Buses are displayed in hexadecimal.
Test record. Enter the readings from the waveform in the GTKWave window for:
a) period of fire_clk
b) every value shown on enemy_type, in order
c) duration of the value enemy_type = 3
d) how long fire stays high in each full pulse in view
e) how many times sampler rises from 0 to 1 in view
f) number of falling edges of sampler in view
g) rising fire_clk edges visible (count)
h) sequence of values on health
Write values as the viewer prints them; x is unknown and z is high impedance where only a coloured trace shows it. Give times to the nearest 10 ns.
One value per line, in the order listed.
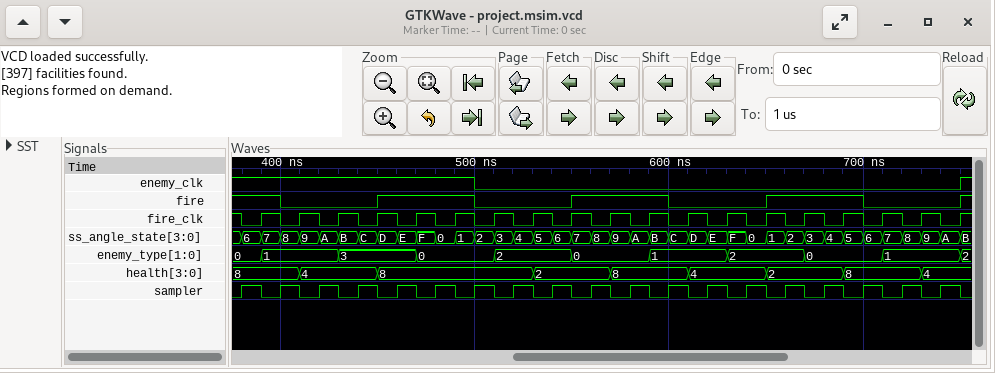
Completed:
20 ns
0, 1, 3, 0, 2, 0, 1, 2, 0, 1, 2
40 ns
50 ns, 50 ns, 50 ns
19
19
19
8, 4, 8, 2, 8, 4, 2, 8, 4
